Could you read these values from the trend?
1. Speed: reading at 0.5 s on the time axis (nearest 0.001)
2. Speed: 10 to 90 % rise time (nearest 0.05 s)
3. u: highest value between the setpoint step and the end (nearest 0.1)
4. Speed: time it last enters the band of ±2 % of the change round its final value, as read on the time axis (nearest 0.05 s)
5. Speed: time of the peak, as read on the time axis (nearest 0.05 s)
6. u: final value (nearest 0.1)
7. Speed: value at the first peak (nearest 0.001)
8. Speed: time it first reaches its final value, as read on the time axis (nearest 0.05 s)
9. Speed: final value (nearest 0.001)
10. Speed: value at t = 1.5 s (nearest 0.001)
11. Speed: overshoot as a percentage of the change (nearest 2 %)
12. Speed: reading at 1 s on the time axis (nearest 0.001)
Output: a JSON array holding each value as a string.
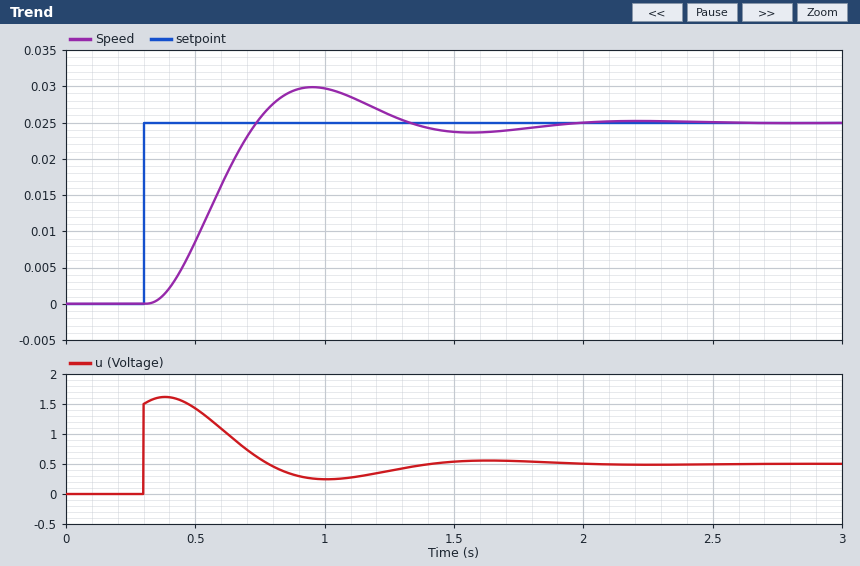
["0.009", "0.30 s", "1.6", "1.85 s", "0.95 s", "0.5", "0.030", "0.75 s", "0.025", "0.024", "20 %", "0.030"]
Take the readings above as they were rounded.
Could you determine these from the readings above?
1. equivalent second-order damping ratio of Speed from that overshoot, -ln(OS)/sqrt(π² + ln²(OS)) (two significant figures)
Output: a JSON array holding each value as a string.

["0.46"]
